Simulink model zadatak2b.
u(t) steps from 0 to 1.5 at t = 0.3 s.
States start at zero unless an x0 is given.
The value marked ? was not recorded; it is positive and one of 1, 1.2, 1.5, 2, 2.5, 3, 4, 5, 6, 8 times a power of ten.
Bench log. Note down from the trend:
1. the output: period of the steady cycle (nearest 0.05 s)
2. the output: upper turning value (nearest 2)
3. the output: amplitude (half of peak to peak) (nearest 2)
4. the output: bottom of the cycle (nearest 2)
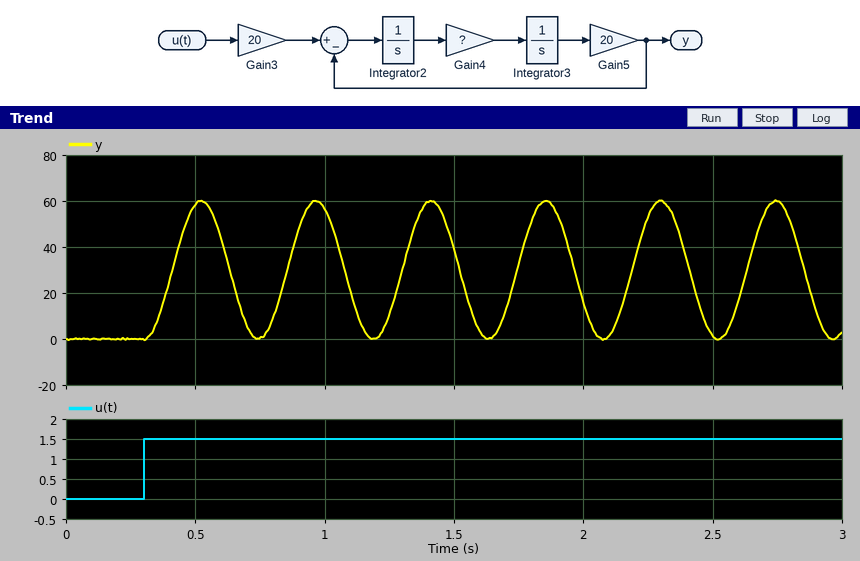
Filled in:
0.45 s
60
30
0
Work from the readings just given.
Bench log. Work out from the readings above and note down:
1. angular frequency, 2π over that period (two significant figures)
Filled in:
14 rad/s
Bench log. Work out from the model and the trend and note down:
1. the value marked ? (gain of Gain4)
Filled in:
10
